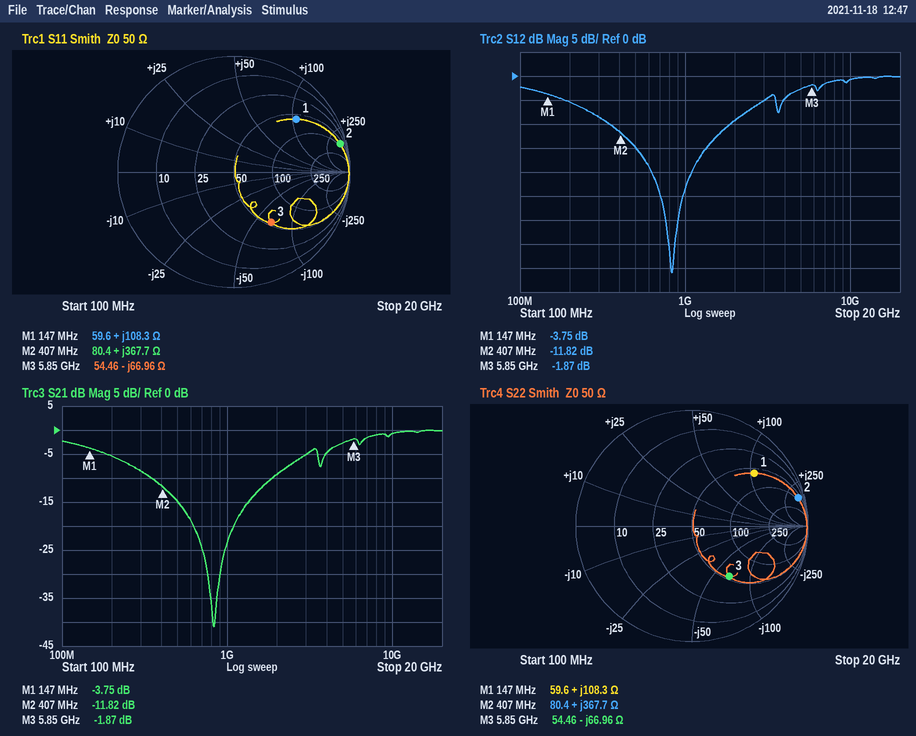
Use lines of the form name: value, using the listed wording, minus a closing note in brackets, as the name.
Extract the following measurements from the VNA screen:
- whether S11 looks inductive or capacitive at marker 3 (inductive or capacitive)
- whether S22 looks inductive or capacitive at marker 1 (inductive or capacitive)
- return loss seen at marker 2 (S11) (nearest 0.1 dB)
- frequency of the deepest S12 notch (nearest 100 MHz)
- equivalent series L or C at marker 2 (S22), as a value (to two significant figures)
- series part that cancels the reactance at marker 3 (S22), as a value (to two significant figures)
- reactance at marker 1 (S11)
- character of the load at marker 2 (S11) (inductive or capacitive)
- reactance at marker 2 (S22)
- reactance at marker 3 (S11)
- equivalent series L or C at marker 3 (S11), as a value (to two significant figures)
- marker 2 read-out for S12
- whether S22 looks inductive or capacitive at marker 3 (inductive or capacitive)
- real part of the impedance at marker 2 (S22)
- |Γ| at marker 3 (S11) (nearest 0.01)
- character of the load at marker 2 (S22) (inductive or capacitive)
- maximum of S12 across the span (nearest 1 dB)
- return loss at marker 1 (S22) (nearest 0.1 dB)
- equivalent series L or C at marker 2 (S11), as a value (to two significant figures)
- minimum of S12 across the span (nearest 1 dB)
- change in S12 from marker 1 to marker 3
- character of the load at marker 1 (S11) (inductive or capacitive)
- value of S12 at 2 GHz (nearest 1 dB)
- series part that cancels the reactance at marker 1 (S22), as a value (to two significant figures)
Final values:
whether S11 looks inductive or capacitive at marker 3: capacitive
whether S22 looks inductive or capacitive at marker 1: inductive
return loss seen at marker 2 (S11): 0.5 dB
frequency of the deepest S12 notch: 800 MHz
equivalent series L or C at marker 2 (S22), as a value: 140 nH
series part that cancels the reactance at marker 3 (S22), as a value: 1.8 nH
reactance at marker 1: +108.3 Ω
character of the load at marker 2 (S11): inductive
reactance at marker 2: +367.7 Ω
reactance at marker 3: -66.96 Ω
equivalent series L or C at marker 3 (S11), as a value: 410 fF
marker 2 read-out for S12: -11.82 dB
whether S22 looks inductive or capacitive at marker 3: capacitive
real part of the impedance at marker 2: 80.4 Ω
|Γ| at marker 3 (S11): 0.54
character of the load at marker 2 (S22): inductive
maximum of S12 across the span: 0 dB
return loss at marker 1 (S22): 3.0 dB
equivalent series L or C at marker 2 (S11), as a value: 140 nH
minimum of S12 across the span: -41 dB
change in S12 from marker 1 to marker 3: 1.88 dB
character of the load at marker 1 (S11): inductive
value of S12 at 2 GHz: -9 dB
series part that cancels the reactance at marker 1 (S22), as a value: 10.0 pF
